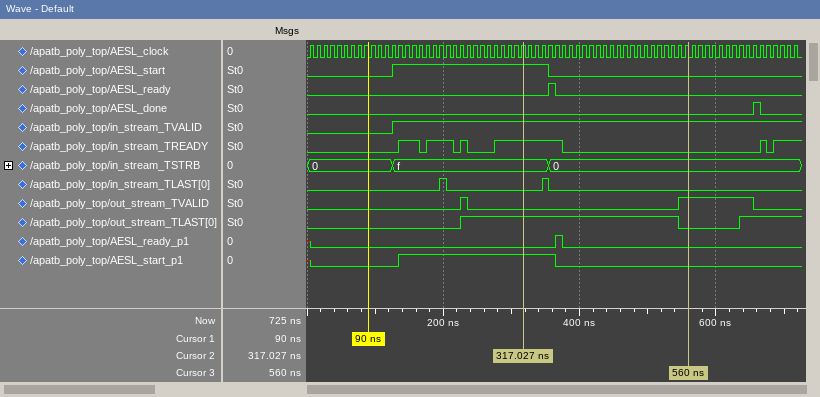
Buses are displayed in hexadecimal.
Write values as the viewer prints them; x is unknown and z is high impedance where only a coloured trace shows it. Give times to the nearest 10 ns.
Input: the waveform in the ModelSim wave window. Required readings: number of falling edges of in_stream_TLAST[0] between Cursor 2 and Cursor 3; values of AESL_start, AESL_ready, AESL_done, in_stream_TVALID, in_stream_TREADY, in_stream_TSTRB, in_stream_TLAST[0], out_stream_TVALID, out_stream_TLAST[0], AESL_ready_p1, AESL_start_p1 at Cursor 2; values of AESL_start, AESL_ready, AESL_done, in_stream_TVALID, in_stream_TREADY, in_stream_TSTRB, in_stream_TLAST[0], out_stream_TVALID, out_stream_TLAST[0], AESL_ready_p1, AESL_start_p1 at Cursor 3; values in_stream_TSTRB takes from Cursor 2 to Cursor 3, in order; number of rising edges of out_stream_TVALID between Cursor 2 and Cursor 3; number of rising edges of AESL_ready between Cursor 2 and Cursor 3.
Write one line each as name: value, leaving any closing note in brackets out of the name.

number of falling edges of in_stream_TLAST[0] between Cursor 2 and Cursor 3: 1
values of AESL_start, AESL_ready, AESL_done, in_stream_TVALID, in_stream_TREADY, in_stream_TSTRB, in_stream_TLAST[0], out_stream_TVALID, out_stream_TLAST[0], AESL_ready_p1, AESL_start_p1 at Cursor 2: AESL_start=1, AESL_ready=0, AESL_done=0, in_stream_TVALID=1, in_stream_TREADY=1, in_stream_TSTRB=f, in_stream_TLAST[0]=0, out_stream_TVALID=0, out_stream_TLAST[0]=1, AESL_ready_p1=0, AESL_start_p1=1
values of AESL_start, AESL_ready, AESL_done, in_stream_TVALID, in_stream_TREADY, in_stream_TSTRB, in_stream_TLAST[0], out_stream_TVALID, out_stream_TLAST[0], AESL_ready_p1, AESL_start_p1 at Cursor 3: AESL_start=0, AESL_ready=0, AESL_done=0, in_stream_TVALID=1, in_stream_TREADY=0, in_stream_TSTRB=0, in_stream_TLAST[0]=0, out_stream_TVALID=1, out_stream_TLAST[0]=0, AESL_ready_p1=0, AESL_start_p1=0
values in_stream_TSTRB takes from Cursor 2 to Cursor 3, in order: f, 0
number of rising edges of out_stream_TVALID between Cursor 2 and Cursor 3: 1
number of rising edges of AESL_ready between Cursor 2 and Cursor 3: 1
